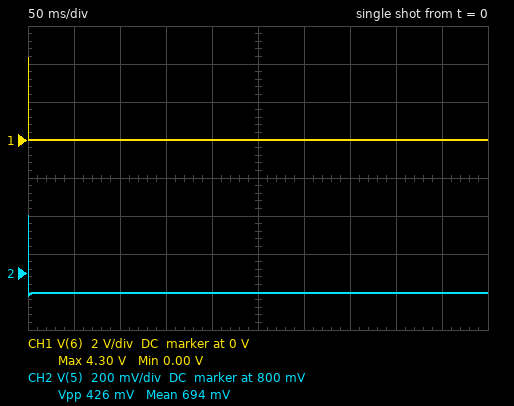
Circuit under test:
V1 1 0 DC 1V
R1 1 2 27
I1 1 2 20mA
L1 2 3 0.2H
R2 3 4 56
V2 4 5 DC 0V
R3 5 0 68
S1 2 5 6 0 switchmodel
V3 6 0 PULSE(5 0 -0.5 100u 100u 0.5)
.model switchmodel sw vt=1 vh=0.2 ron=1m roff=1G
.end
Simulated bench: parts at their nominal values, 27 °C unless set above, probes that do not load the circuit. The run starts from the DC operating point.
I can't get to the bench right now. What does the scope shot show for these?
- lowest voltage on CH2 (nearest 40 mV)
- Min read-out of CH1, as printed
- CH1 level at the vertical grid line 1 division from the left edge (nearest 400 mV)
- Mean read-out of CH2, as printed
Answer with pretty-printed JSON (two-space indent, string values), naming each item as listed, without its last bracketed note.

{
  "lowest voltage on CH2": "680 mV",
  "Min read-out of CH1, as printed": "0.00 V",
  "CH1 level at the vertical grid line 1 division from the left edge": "0 V",
  "Mean read-out of CH2, as printed": "694 mV"
}
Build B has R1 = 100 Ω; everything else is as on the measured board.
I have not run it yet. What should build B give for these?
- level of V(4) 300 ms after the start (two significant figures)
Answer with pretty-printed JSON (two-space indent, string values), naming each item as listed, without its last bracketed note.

{
  "level of V(4) 300 ms after the start": "910 mV"
}
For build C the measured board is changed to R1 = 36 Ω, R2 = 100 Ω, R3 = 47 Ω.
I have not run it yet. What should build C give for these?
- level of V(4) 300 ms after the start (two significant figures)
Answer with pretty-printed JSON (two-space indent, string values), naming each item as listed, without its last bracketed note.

{
  "level of V(4) 300 ms after the start": "440 mV"
}
